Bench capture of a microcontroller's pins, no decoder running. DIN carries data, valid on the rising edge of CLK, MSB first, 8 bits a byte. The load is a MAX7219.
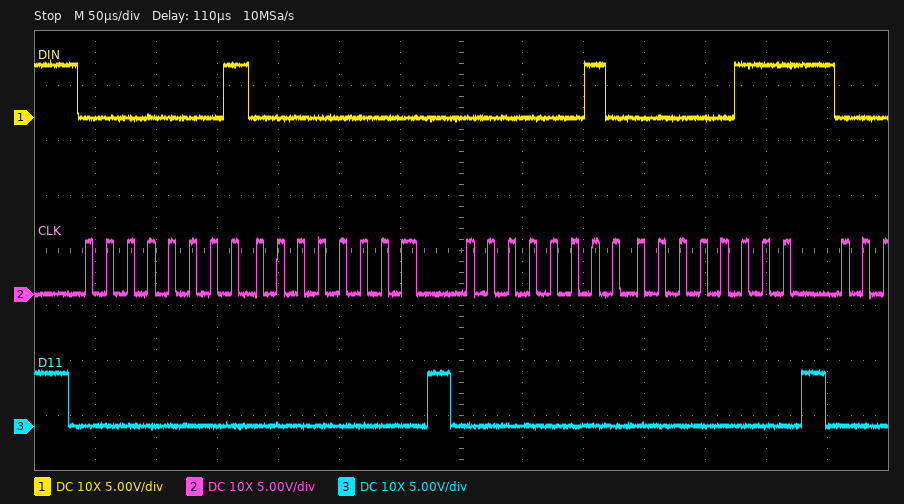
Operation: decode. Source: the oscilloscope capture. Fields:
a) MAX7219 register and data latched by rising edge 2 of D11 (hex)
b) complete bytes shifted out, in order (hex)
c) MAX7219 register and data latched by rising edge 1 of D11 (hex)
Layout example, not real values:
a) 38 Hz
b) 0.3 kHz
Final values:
a) register 0x2, data 0x07
b) 01 00 02 07
c) register 0x1, data 0x00
